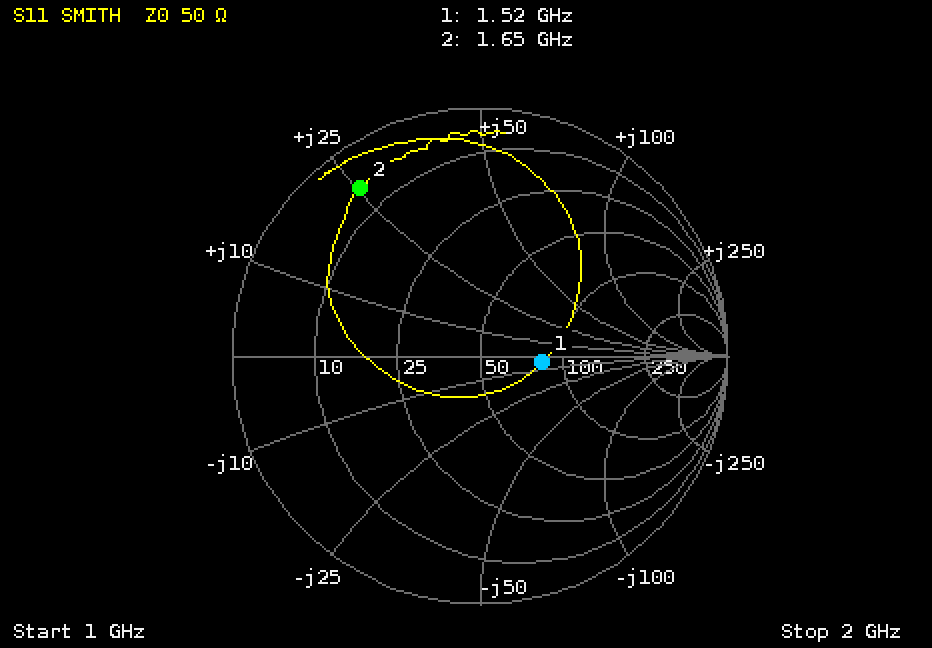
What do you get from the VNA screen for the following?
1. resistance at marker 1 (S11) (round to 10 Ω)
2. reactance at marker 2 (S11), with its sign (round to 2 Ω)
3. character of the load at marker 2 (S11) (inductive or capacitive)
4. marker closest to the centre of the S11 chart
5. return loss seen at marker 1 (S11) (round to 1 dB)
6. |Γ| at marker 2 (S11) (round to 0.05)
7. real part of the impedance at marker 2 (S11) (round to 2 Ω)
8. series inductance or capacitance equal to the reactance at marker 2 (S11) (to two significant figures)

80 Ω
+26 Ω
inductive
marker 1
12 dB
0.85
6 Ω
2.5 nH
